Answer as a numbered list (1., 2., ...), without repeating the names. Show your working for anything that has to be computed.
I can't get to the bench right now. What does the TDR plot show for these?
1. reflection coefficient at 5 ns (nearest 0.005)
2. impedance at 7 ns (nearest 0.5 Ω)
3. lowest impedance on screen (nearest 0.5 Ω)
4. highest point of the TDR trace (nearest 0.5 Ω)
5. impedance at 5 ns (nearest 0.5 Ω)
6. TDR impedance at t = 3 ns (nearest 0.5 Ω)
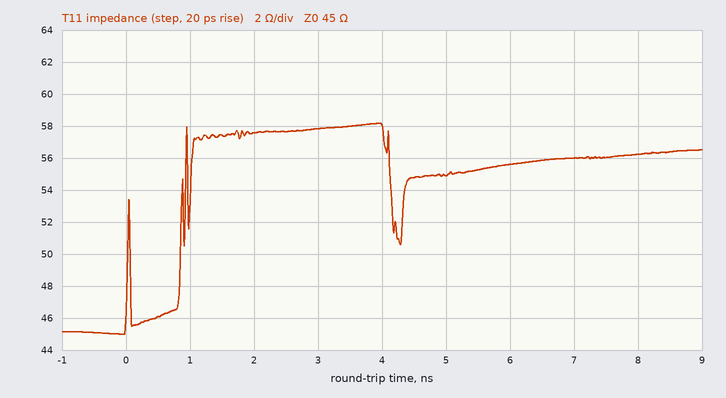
1. (55 − 45)/(55 + 45) ≈ +0.100
2. 56.0 Ω
3. 45.0 Ω
4. 58.0 Ω
5. 55.0 Ω
6. 58.0 Ω
